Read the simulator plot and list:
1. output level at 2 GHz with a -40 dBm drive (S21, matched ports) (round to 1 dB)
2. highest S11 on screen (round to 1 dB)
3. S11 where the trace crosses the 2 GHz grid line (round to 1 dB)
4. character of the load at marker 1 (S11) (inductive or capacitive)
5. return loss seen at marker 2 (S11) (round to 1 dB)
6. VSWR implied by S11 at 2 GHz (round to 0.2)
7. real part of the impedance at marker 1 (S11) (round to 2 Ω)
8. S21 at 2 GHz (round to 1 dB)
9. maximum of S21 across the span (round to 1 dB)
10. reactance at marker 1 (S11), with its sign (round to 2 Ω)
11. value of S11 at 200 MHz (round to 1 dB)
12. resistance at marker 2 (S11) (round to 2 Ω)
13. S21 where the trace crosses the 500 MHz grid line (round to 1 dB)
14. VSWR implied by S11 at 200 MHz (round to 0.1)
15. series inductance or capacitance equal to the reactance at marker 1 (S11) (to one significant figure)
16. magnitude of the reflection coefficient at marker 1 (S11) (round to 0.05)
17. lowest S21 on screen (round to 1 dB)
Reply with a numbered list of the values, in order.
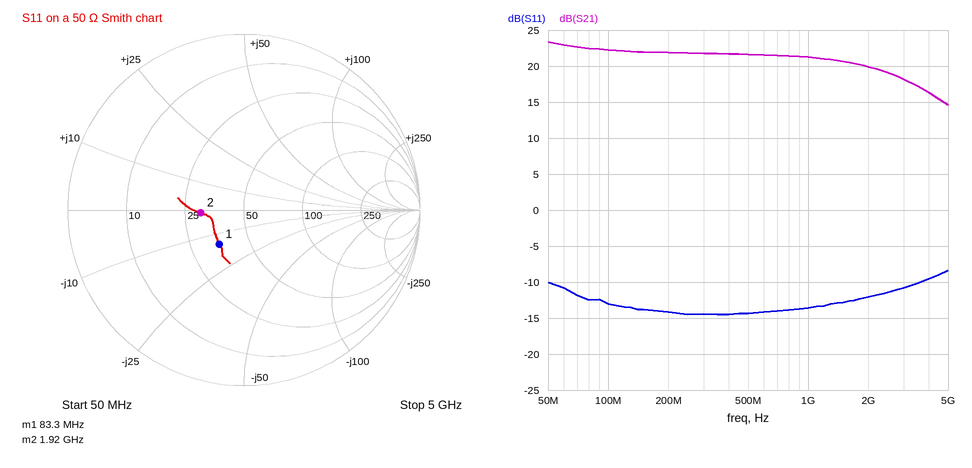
1. -20 dBm
2. -8 dB
3. -12 dB
4. capacitive
5. 12 dB
6. 1.6
7. 36 Ω
8. 20 dB
9. 23 dB
10. -14 Ω
11. -14 dB
12. 30 Ω
13. 22 dB
14. 1.5
15. 100 pF
16. 0.25
17. 15 dB
